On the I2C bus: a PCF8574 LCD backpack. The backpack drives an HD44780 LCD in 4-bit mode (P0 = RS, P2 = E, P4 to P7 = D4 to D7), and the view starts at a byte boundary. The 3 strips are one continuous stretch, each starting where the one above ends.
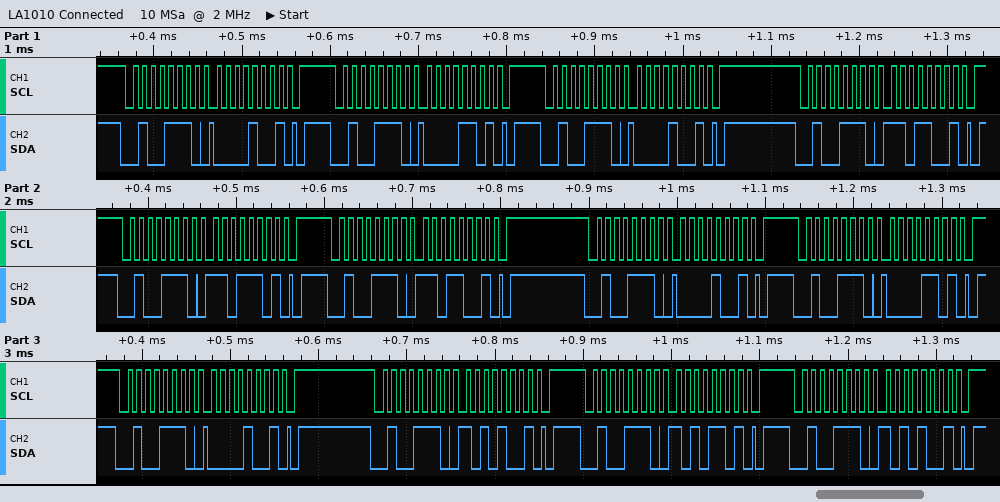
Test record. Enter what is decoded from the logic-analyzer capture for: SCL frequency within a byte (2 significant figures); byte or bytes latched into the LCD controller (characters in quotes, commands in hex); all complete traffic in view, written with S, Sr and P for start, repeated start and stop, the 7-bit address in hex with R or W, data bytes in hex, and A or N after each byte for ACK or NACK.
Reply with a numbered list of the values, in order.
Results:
1. 100 kHz
2. data 0x0D data 0x0A
3. S 27W A 09 A P S 27W A 0D A P S 27W A 09 A P S 27W A D9 A P S 27W A DD A P S 27W A D9 A P S 27W A 09 A P S 27W A 0D A P S 27W A 09 A P S 27W A A9 A P S 27W A AD A P S 27W A A9 A P
